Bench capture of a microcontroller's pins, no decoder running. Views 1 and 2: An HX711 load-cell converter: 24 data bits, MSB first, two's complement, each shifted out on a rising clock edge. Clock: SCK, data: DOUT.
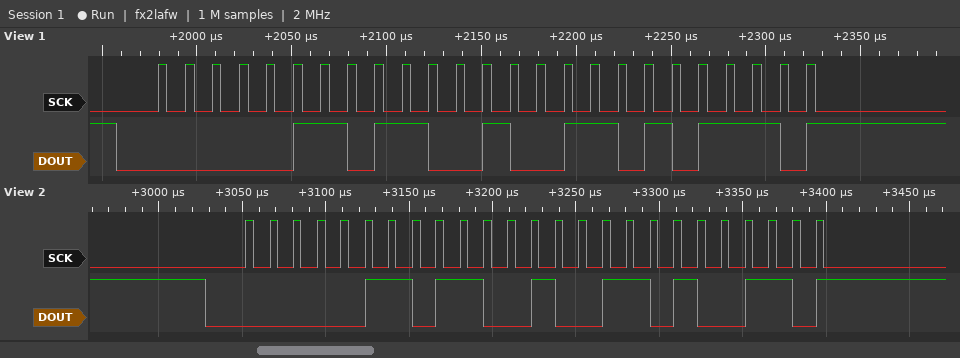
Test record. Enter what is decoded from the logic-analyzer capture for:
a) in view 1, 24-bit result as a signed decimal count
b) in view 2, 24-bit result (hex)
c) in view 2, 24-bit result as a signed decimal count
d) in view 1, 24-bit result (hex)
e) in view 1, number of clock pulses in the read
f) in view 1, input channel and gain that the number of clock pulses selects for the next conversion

444846
0x06C9A6
444838
0x06C9AE
25
channel A, gain 128
